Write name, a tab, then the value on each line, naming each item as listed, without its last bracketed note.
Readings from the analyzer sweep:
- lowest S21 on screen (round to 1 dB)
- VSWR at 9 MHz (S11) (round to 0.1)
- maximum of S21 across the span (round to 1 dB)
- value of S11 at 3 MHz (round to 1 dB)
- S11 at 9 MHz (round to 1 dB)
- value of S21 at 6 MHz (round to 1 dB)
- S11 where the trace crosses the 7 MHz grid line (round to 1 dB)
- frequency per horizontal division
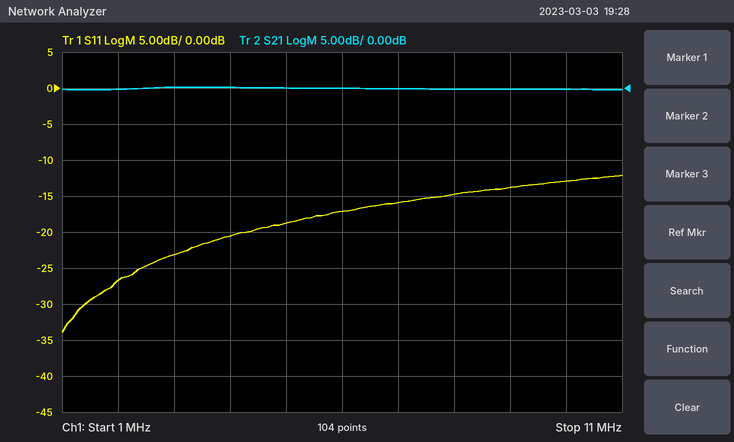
lowest S21 on screen	0 dB
VSWR at 9 MHz (S11)	1.5
maximum of S21 across the span	0 dB
value of S11 at 3 MHz	-23 dB
S11 at 9 MHz	-14 dB
value of S21 at 6 MHz	0 dB
S11 where the trace crosses the 7 MHz grid line	-16 dB
frequency per horizontal division	1 MHz
